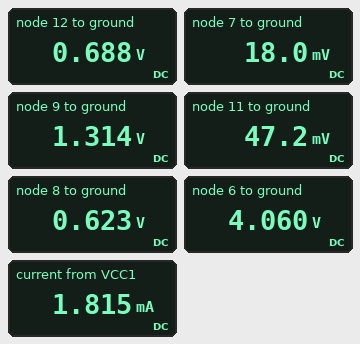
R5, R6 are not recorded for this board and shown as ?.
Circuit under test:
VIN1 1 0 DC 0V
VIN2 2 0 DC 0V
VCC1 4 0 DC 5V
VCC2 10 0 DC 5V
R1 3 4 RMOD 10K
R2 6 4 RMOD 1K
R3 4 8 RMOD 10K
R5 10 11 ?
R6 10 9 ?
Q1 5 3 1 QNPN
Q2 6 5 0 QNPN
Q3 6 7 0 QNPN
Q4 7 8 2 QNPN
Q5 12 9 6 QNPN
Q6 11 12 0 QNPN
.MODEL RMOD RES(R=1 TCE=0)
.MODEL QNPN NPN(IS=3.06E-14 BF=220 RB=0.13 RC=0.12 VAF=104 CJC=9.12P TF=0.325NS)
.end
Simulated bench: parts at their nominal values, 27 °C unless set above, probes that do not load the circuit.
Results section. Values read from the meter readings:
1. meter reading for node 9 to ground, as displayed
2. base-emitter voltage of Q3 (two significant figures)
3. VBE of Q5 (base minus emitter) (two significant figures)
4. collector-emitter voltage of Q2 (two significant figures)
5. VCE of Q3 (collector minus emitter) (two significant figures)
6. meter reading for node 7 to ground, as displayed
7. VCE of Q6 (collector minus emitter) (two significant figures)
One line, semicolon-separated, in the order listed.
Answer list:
1.314 V; 18 mV; -2.7 V; 4.1 V; 4.1 V; 18.0 mV; 47 mV
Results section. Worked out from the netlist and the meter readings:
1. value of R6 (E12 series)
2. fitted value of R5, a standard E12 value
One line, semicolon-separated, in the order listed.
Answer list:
3.9 kΩ; 680 Ω
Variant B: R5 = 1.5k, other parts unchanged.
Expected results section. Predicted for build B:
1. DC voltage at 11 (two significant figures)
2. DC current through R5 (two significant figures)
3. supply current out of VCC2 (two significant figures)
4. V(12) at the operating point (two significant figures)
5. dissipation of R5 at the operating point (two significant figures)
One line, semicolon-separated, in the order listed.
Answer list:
35 mV; 3.3 mA; 4.3 mA; 680 mV; 16 mW
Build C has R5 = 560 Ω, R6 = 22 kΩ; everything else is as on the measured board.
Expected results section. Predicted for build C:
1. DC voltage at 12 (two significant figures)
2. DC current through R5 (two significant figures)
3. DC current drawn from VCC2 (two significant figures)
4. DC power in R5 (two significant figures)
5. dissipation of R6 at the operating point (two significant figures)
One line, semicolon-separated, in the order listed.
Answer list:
680 mV; 8.8 mA; 8.9 mA; 43 mW; 630 µW
